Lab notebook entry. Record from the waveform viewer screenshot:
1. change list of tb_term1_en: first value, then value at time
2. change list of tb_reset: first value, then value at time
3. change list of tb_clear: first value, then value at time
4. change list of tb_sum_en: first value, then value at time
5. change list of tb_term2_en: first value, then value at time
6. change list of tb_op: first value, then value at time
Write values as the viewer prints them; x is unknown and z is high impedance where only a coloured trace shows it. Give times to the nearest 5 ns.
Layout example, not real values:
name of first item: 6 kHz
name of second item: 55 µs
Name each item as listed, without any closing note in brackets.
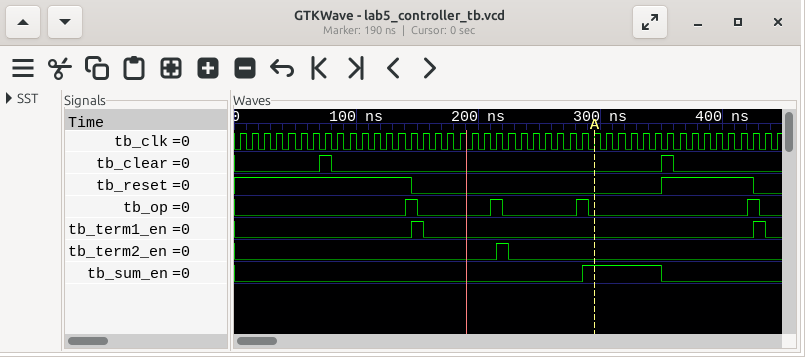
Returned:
change list of tb_term1_en: first value, then value at time: 0, 1 at 145 ns, 0 at 155 ns, 1 at 425 ns, 0 at 435 ns
change list of tb_reset: first value, then value at time: 1, 0 at 145 ns, 1 at 350 ns, 0 at 425 ns
change list of tb_clear: first value, then value at time: 0, 1 at 70 ns, 0 at 80 ns, 1 at 350 ns, 0 at 360 ns
change list of tb_sum_en: first value, then value at time: 0, 1 at 285 ns, 0 at 350 ns
change list of tb_term2_en: first value, then value at time: 0, 1 at 215 ns, 0 at 225 ns
change list of tb_op: first value, then value at time: 0, 1 at 140 ns, 0 at 150 ns, 1 at 210 ns, 0 at 220 ns, 1 at 280 ns, 0 at 290 ns, 1 at 420 ns, 0 at 430 ns
